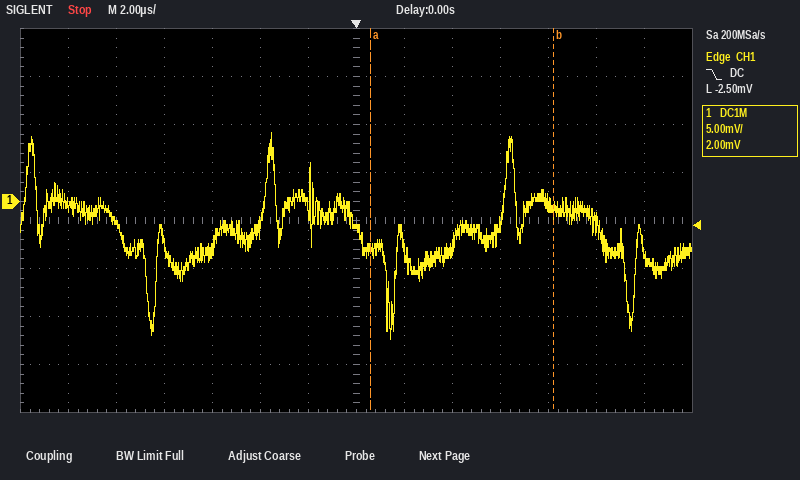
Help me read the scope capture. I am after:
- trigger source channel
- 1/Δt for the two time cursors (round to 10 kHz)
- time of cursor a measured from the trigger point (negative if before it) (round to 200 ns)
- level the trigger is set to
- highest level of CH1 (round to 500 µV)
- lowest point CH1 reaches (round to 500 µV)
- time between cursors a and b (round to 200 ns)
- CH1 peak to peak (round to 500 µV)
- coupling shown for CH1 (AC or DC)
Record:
CH1
130 kHz
+600 ns
-2.50 mV
7.0 mV
-14.5 mV
7.6 µs
21.5 mV
DC
